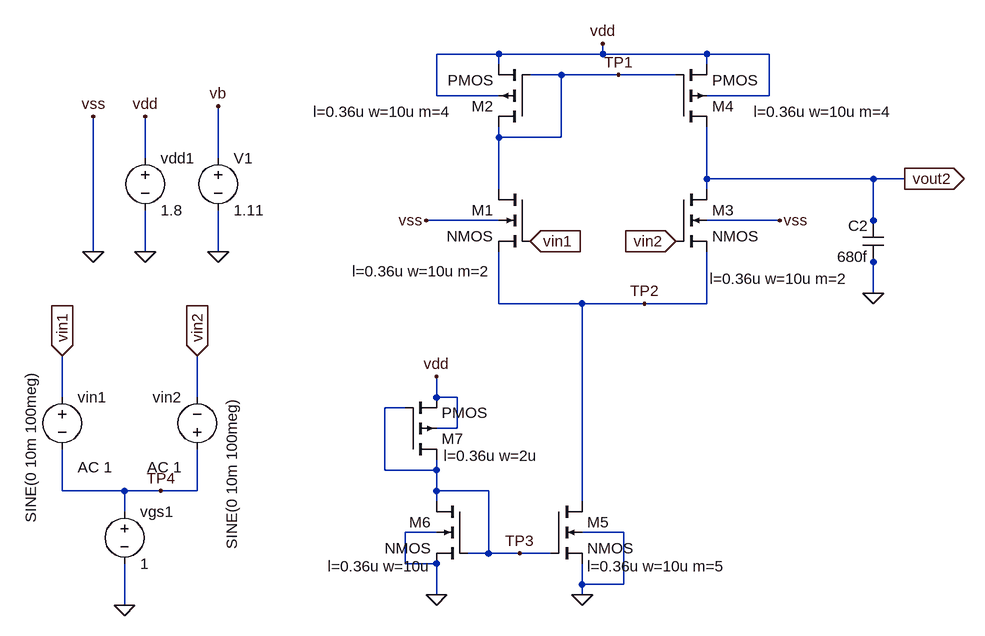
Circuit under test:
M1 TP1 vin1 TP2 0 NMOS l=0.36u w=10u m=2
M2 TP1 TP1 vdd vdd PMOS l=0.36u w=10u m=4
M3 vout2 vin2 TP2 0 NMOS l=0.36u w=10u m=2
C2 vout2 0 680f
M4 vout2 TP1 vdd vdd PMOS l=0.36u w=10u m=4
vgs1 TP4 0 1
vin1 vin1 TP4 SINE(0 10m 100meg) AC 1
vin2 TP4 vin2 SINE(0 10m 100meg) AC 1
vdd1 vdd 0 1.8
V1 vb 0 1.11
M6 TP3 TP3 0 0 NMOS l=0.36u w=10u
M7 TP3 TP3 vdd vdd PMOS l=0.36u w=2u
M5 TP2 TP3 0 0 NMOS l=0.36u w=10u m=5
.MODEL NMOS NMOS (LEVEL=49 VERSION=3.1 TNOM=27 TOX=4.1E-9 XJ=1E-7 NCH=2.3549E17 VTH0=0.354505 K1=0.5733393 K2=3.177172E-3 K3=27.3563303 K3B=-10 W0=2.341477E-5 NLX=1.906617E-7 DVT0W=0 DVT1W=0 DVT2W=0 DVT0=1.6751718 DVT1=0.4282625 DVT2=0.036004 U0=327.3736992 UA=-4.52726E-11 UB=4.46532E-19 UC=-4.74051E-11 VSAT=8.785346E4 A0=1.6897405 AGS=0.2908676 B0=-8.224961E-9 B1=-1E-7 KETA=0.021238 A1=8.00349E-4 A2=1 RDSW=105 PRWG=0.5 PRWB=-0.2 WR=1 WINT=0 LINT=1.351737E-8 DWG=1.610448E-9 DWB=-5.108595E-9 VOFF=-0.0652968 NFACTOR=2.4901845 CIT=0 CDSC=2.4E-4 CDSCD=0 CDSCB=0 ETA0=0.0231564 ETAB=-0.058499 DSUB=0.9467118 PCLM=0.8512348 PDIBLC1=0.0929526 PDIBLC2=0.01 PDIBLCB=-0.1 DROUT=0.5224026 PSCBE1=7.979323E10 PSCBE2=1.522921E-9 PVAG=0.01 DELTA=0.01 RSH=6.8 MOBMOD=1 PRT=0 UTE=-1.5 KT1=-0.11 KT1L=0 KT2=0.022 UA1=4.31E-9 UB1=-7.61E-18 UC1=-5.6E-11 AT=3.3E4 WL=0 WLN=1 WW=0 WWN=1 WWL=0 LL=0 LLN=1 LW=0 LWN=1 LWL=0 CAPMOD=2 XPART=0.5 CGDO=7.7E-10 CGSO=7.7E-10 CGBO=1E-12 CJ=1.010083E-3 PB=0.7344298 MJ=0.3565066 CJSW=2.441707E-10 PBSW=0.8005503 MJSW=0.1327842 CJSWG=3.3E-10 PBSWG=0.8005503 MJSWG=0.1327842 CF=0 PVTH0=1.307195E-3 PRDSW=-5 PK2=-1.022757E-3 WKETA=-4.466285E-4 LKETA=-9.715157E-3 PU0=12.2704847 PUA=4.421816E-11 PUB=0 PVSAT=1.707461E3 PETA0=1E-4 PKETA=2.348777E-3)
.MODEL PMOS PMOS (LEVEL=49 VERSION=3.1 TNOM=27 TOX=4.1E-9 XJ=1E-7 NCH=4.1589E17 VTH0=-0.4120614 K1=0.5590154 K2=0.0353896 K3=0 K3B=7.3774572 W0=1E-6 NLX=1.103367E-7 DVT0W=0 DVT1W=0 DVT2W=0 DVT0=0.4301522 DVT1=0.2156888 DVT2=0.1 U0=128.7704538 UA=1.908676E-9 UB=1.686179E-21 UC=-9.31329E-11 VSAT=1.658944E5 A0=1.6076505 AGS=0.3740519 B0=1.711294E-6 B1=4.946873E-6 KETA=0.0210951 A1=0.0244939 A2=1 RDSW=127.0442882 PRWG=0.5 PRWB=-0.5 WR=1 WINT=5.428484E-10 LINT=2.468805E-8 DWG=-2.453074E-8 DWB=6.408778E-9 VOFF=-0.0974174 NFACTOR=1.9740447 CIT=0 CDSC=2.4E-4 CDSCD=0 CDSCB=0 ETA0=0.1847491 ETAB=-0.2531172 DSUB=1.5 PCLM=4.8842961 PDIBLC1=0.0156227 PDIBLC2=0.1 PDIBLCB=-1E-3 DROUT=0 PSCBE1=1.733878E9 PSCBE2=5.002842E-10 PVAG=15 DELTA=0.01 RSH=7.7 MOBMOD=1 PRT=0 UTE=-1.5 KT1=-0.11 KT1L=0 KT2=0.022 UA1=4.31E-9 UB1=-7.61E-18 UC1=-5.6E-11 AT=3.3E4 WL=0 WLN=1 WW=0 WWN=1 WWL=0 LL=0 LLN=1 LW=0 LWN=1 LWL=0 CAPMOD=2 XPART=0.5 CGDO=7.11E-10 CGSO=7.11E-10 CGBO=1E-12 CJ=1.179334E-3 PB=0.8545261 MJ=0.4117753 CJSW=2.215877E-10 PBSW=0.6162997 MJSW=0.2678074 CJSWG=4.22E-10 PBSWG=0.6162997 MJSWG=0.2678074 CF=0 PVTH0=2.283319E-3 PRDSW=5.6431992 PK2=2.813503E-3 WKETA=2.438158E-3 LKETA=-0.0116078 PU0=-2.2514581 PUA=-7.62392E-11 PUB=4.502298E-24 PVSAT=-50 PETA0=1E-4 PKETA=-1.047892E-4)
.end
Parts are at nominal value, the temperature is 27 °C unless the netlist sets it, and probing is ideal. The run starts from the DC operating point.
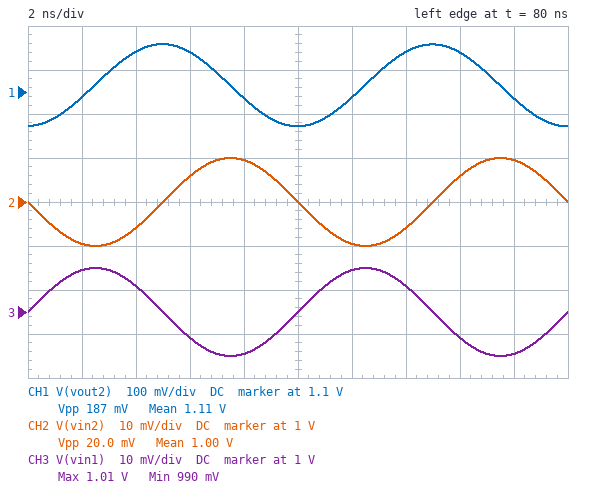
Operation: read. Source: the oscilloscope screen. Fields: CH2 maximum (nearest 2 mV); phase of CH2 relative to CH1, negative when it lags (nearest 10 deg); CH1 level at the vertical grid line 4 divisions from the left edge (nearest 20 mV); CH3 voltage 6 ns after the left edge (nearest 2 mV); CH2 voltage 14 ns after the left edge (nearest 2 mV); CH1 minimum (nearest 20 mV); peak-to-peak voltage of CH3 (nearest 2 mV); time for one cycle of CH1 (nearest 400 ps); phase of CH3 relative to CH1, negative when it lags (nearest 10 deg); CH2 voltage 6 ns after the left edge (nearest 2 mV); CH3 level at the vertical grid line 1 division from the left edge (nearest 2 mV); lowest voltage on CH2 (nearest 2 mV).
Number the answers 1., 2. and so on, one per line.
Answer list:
1. 1.010 V
2. -90 deg
3. 1.08 V
4. 994 mV
5. 994 mV
6. 1.02 V
7. 20 mV
8. 10.0 ns
9. 90 deg
10. 1.006 V
11. 1.010 V
12. 990 mV
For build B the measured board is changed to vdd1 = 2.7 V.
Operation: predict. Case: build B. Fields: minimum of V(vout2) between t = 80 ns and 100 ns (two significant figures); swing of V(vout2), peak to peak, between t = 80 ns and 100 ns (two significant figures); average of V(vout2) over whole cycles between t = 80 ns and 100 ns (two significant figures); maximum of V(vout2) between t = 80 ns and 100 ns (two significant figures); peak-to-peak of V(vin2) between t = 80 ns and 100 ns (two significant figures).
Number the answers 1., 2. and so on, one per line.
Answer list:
1. 1.7 V
2. 300 mV
3. 1.8 V
4. 2.0 V
5. 20 mV
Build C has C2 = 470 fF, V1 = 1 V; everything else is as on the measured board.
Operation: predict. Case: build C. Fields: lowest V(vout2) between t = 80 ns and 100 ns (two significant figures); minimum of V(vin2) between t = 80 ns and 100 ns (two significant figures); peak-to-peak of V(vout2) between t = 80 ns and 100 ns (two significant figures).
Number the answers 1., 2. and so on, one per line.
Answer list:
1. 990 mV
2. 990 mV
3. 260 mV
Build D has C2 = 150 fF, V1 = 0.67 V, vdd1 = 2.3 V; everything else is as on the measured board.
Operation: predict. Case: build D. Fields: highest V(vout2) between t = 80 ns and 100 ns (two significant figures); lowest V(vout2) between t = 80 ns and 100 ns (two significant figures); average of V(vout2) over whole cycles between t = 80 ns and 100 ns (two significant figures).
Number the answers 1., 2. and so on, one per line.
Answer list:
1. 1.9 V
2. 1.1 V
3. 1.5 V
